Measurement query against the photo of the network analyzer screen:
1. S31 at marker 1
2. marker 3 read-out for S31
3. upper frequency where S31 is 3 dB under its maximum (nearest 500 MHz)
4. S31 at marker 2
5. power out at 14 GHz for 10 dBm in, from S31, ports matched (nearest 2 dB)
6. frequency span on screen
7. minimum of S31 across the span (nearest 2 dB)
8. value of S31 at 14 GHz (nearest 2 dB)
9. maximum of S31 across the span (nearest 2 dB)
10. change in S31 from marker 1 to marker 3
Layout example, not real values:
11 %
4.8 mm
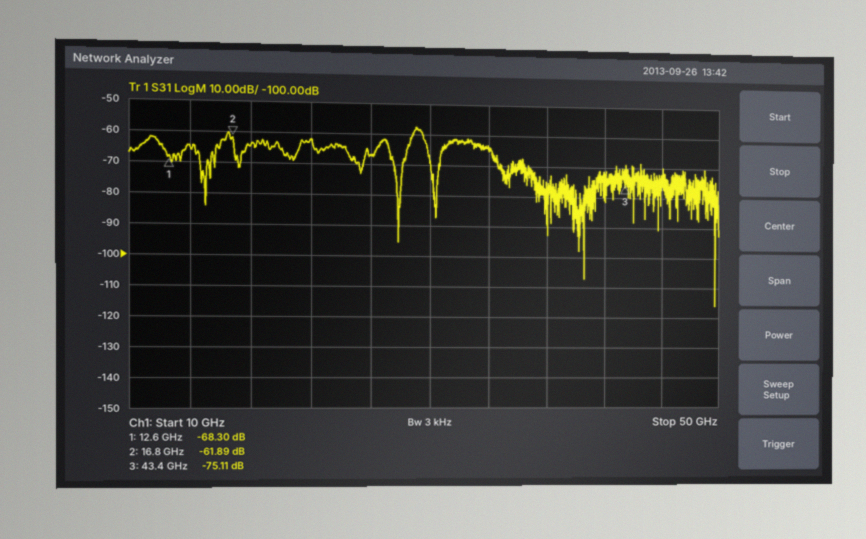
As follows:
-68.30 dB
-75.11 dB
29.5 GHz
-61.89 dB
-56 dBm
40 GHz
-116 dB
-66 dB
-58 dB
-6.81 dB
